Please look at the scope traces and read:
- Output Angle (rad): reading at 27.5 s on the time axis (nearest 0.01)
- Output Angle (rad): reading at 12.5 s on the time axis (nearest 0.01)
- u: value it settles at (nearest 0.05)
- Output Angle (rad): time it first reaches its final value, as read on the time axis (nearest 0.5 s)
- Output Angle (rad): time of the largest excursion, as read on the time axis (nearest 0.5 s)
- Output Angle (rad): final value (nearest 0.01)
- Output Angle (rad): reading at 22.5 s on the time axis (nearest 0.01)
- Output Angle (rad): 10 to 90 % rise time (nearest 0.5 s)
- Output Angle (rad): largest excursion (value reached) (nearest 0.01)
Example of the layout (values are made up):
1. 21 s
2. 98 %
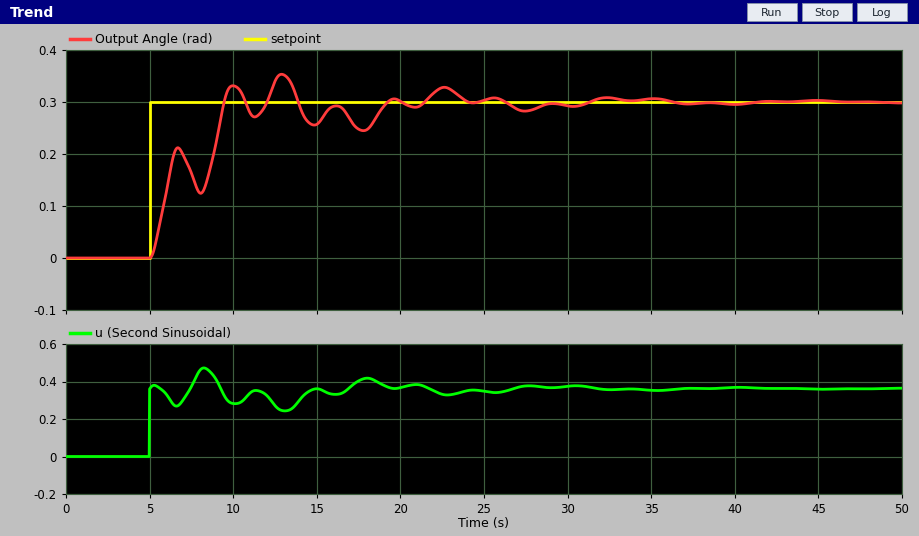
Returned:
1. 0.28
2. 0.34
3. 0.35
4. 9.5 s
5. 13.0 s
6. 0.30
7. 0.33
8. 4.0 s
9. 0.35
